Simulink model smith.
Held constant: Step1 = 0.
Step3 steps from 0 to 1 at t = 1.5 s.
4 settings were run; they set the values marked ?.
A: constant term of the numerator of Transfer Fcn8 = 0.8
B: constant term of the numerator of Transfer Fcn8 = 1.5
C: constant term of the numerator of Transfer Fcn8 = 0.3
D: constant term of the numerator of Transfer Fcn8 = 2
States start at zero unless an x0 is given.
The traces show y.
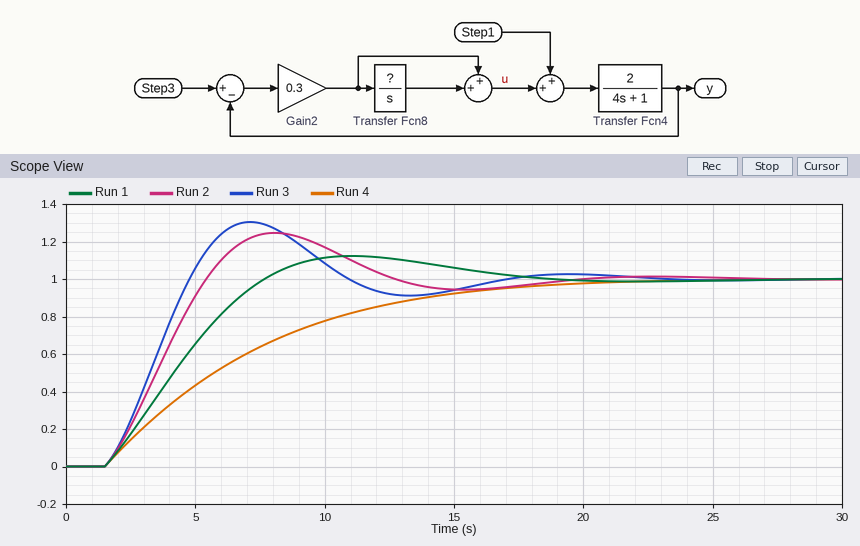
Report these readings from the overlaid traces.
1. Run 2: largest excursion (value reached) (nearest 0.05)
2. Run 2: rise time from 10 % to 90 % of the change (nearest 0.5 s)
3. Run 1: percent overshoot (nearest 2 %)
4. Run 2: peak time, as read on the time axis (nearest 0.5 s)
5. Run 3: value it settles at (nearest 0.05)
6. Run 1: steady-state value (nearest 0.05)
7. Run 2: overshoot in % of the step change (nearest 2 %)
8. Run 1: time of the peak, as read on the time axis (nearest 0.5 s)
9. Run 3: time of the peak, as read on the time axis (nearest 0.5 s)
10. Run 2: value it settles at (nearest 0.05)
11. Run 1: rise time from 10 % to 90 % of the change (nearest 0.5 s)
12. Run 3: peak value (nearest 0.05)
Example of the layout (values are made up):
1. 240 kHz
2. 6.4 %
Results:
1. 1.25
2. 3.0 s
3. 12 %
4. 8.0 s
5. 1.00
6. 1.00
7. 24 %
8. 11.0 s
9. 7.0 s
10. 1.00
11. 4.5 s
12. 1.30
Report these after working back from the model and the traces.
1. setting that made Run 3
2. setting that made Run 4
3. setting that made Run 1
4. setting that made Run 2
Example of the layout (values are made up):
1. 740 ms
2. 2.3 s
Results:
1. D
2. C
3. A
4. B
